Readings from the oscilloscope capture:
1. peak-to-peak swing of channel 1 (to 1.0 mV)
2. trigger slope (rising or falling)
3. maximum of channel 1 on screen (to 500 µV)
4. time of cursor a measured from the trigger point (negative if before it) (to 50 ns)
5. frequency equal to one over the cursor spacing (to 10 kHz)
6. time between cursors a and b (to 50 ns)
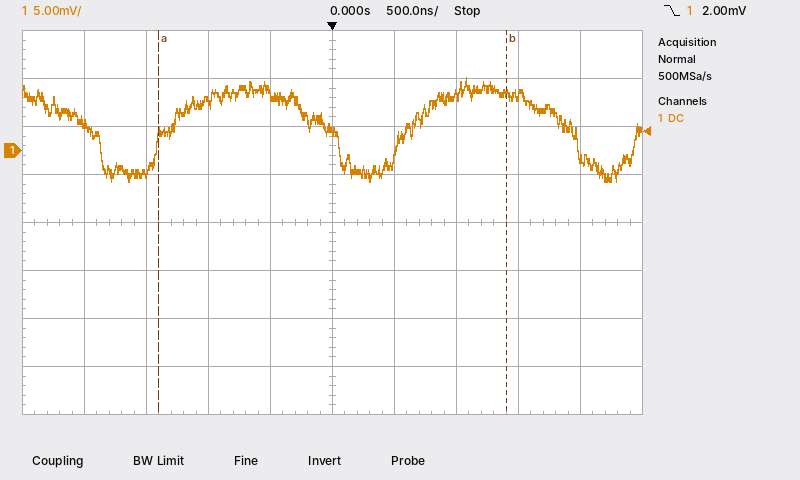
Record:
11.0 mV
falling
7.5 mV
-1.40 µs
360 kHz
2.80 µs
